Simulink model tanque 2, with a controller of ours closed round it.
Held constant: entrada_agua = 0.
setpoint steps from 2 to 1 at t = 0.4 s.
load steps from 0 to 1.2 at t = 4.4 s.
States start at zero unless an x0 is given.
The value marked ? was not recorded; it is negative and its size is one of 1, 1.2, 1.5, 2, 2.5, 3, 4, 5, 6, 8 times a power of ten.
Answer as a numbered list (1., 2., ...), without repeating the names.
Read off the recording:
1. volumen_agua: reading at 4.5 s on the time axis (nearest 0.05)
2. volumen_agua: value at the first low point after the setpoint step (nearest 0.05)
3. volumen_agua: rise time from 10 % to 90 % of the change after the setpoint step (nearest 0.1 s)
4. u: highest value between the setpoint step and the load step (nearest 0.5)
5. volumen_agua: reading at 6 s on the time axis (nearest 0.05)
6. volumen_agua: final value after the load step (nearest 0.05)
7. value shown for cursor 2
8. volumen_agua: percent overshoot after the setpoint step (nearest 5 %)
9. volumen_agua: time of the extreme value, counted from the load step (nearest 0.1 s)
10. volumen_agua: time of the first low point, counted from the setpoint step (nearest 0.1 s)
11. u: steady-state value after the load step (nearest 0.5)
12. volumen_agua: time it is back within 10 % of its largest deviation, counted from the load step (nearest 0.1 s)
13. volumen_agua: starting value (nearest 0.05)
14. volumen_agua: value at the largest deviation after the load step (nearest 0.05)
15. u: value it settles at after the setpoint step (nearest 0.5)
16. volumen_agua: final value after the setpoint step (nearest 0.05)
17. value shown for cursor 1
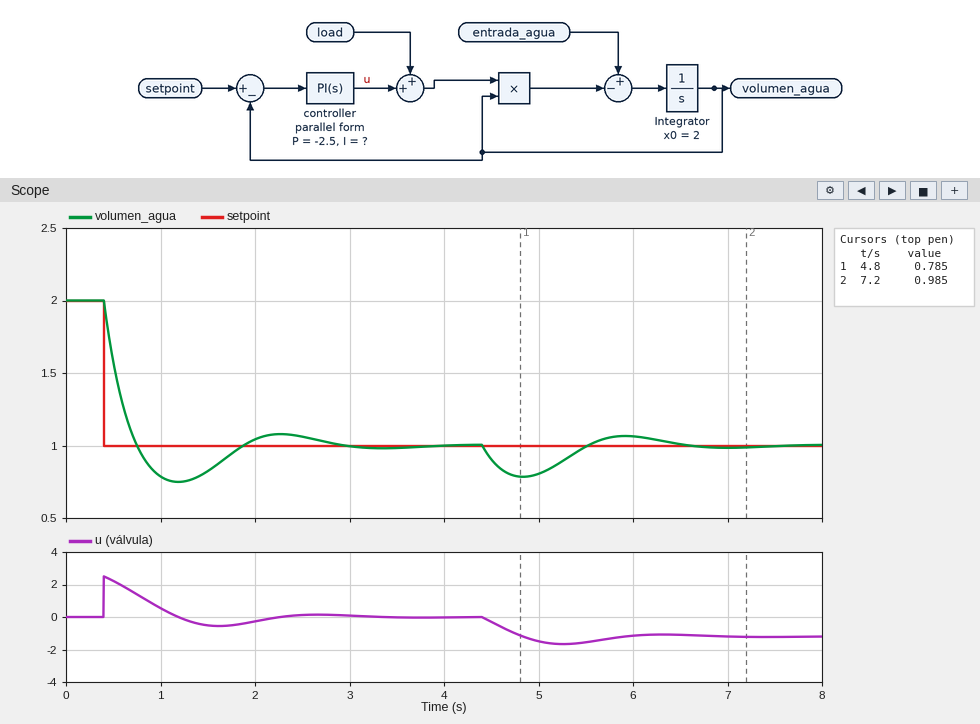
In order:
1. 0.90
2. 0.75
3. 0.3 s
4. 2.5
5. 1.05
6. 1.00
7. 0.985
8. 25 %
9. 0.4 s
10. 0.8 s
11. -1.0
12. 2.0 s
13. 2.00
14. 0.80
15. 0.0
16. 1.00
17. 0.785
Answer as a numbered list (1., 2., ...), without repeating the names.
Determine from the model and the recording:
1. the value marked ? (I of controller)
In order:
1. -10
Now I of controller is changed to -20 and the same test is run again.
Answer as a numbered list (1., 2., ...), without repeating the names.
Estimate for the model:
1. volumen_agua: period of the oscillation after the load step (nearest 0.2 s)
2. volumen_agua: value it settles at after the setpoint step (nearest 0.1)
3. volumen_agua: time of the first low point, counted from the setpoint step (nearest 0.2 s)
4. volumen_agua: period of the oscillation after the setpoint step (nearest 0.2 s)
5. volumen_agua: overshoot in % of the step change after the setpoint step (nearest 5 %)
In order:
1. 1.4 s
2. 1.0
3. 0.6 s
4. 1.4 s
5. 30 %
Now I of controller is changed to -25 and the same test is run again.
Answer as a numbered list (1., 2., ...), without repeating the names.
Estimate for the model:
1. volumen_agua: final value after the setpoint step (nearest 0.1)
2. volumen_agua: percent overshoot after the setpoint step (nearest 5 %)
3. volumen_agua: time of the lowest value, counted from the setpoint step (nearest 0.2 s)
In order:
1. 1.0
2. 35 %
3. 0.6 s
